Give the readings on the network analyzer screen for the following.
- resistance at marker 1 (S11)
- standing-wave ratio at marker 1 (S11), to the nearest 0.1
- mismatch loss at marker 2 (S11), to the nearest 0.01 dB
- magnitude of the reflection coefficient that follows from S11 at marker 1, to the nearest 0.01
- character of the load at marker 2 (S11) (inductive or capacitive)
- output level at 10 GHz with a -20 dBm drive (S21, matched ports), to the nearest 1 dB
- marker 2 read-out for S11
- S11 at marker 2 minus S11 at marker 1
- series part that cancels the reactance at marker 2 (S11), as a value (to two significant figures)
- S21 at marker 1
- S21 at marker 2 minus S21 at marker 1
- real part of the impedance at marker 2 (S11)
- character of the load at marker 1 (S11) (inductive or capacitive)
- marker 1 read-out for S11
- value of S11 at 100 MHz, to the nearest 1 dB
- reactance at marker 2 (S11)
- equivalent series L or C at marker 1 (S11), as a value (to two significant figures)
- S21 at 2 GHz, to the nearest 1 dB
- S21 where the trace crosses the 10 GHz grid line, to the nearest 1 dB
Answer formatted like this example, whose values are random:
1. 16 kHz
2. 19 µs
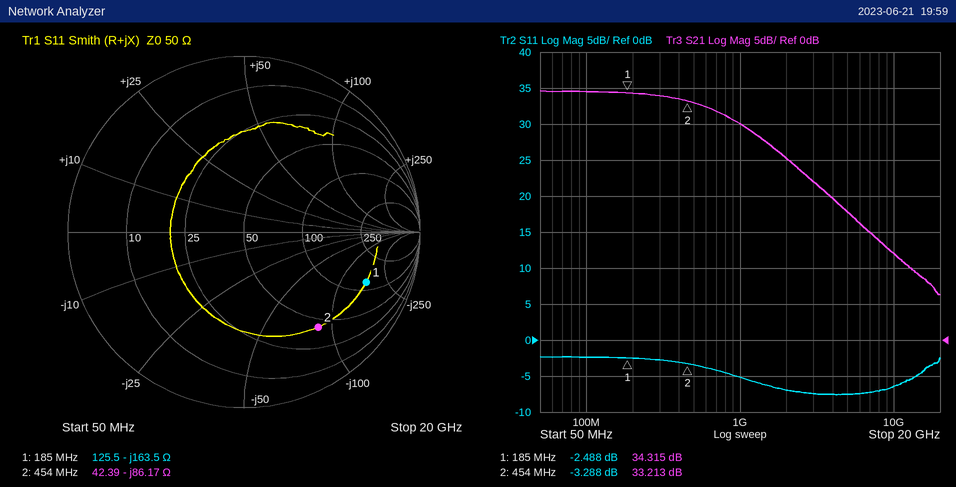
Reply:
1. 125.5 Ω
2. 7.0
3. 2.75 dB
4. 0.75
5. capacitive
6. -8 dBm
7. -3.288 dB
8. -0.800 dB
9. 30 nH
10. 34.315 dB
11. -1.102 dB
12. 42.39 Ω
13. capacitive
14. -2.488 dB
15. -2 dB
16. -86.17 Ω
17. 5.3 pF
18. 25 dB
19. 12 dB
